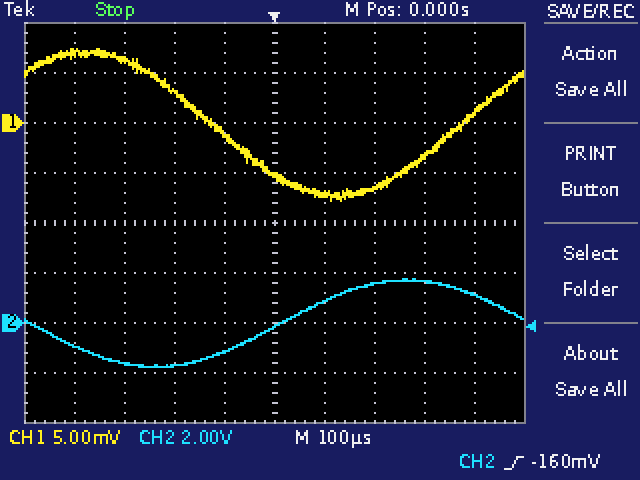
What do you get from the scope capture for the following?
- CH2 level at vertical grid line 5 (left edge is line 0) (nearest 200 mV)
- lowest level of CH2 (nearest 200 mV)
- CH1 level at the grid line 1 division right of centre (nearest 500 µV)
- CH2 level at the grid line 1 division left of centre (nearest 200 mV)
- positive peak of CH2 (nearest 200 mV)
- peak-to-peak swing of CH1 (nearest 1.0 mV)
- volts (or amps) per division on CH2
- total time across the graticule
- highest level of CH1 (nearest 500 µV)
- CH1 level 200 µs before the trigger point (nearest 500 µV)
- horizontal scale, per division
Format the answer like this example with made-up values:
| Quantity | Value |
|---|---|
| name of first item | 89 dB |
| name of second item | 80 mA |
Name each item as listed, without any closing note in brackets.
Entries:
| Quantity | Value |
|---|---|
| CH2 level at vertical grid line 5 (left edge is line 0) | -200 mV |
| lowest level of CH2 | -1.8 V |
| CH1 level at the grid line 1 division right of centre | -7.0 mV |
| CH2 level at the grid line 1 division left of centre | -1.2 V |
| positive peak of CH2 | 1.8 V |
| peak-to-peak swing of CH1 | 15.0 mV |
| volts (or amps) per division on CH2 | 2 V |
| total time across the graticule | 1 ms |
| highest level of CH1 | 7.5 mV |
| CH1 level 200 µs before the trigger point | 3.0 mV |
| horizontal scale, per division | 100 µs |
